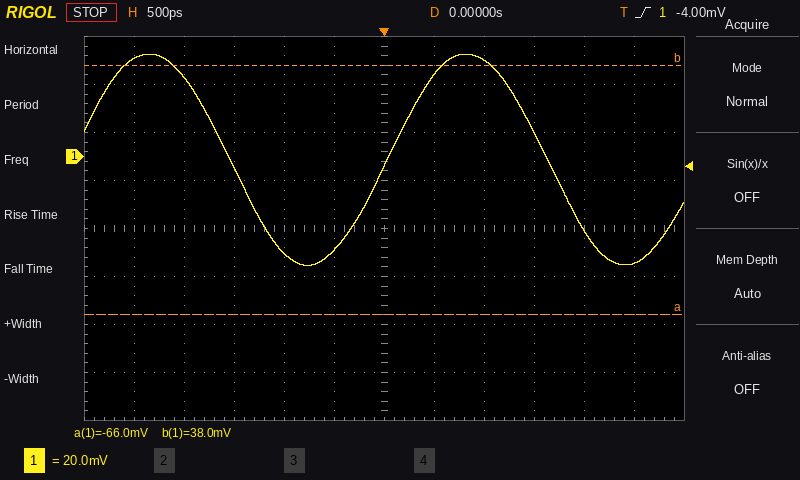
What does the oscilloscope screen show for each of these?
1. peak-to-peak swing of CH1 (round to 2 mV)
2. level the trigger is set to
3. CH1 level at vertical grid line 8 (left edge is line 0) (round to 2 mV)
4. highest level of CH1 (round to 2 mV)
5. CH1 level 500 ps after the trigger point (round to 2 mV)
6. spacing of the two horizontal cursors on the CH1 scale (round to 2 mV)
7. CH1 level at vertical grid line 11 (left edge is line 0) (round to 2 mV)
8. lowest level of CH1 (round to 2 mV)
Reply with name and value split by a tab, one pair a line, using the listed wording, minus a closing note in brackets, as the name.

peak-to-peak swing of CH1	88 mV
level the trigger is set to	-4.00 mV
CH1 level at vertical grid line 8 (left edge is line 0)	40 mV
highest level of CH1	42 mV
CH1 level 500 ps after the trigger point	34 mV
spacing of the two horizontal cursors on the CH1 scale	104 mV
CH1 level at vertical grid line 11 (left edge is line 0)	-44 mV
lowest level of CH1	-46 mV
